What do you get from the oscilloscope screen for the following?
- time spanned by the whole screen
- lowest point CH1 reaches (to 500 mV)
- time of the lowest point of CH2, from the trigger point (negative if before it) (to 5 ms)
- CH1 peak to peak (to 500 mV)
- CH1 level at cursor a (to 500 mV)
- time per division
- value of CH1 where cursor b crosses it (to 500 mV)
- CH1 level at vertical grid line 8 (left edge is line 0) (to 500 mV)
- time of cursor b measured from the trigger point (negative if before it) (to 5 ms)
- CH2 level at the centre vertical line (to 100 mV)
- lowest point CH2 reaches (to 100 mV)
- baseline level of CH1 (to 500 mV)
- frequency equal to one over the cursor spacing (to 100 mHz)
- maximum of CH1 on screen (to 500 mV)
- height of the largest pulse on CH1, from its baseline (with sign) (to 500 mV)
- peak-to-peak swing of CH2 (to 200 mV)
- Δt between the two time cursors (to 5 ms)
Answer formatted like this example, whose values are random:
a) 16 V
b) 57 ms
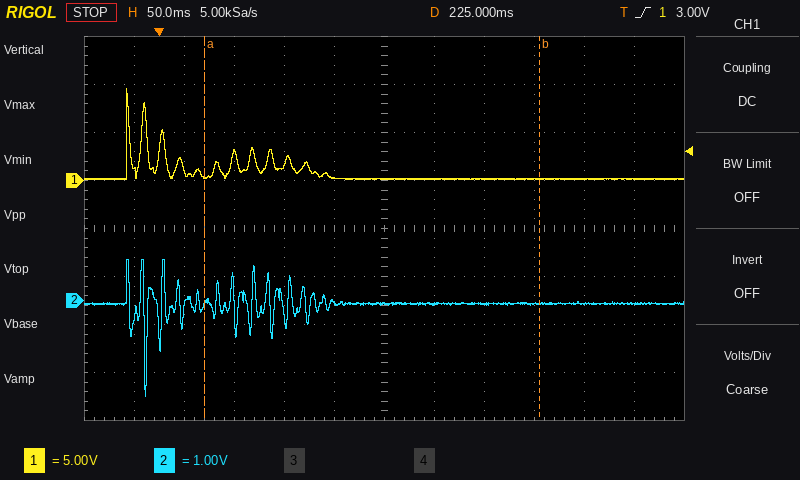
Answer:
a) 600 ms
b) 0.0 V
c) -15 ms
d) 9.5 V
e) 500 mV
f) 50 ms
g) 0.0 V
h) 0.0 V
i) +380 ms
j) -100 mV
k) -2.0 V
l) 0.0 V
m) 3.0 Hz
n) 9.5 V
o) +9.5 V
p) 2.8 V
q) 335 ms
